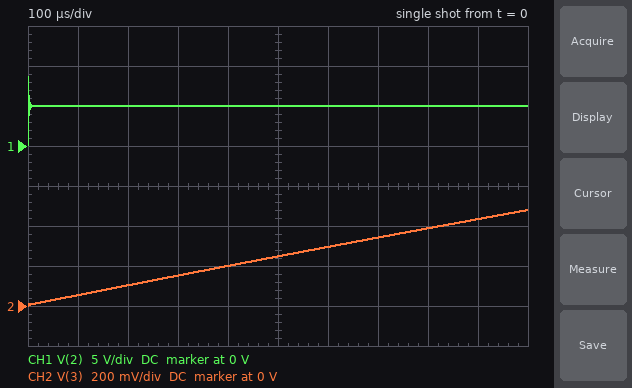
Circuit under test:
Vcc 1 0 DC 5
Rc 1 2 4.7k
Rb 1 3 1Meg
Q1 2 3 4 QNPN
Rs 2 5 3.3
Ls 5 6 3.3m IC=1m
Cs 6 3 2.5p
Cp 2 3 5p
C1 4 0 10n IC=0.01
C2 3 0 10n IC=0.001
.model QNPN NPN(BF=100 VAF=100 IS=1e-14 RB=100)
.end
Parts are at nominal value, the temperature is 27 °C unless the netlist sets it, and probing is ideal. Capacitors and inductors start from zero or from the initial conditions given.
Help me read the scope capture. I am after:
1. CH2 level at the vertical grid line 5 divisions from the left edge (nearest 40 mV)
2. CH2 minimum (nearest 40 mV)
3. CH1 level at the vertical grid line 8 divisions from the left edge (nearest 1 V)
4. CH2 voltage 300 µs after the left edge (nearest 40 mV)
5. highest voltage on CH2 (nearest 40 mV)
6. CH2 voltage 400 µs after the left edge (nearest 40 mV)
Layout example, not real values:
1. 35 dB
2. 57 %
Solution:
1. 240 mV
2. 0 V
3. 5 V
4. 160 mV
5. 480 mV
6. 200 mV
